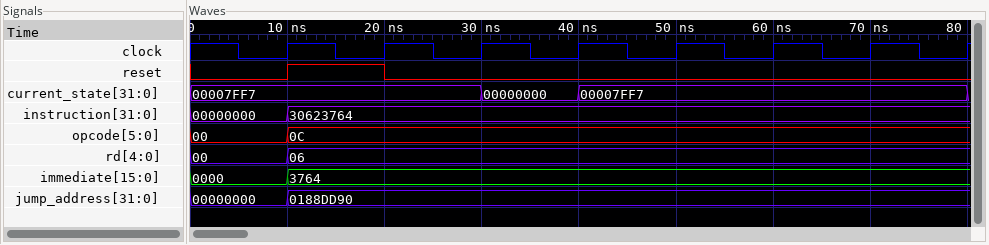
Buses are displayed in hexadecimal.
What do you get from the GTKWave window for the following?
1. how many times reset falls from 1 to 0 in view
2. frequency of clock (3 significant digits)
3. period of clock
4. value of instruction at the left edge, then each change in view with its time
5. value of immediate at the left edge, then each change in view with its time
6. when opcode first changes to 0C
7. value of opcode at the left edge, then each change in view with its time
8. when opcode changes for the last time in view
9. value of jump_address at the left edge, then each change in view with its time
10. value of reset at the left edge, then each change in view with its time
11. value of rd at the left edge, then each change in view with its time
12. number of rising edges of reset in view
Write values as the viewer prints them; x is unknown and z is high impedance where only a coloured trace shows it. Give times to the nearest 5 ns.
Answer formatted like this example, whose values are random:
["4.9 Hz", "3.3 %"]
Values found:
["1", "100 MHz", "10 ns", "00000000, 30623764 at 10 ns", "0000, 3764 at 10 ns", "10 ns", "00, 0C at 10 ns", "10 ns", "00000000, 0188DD90 at 10 ns", "0, 1 at 10 ns, 0 at 20 ns", "00, 06 at 10 ns", "1"]
